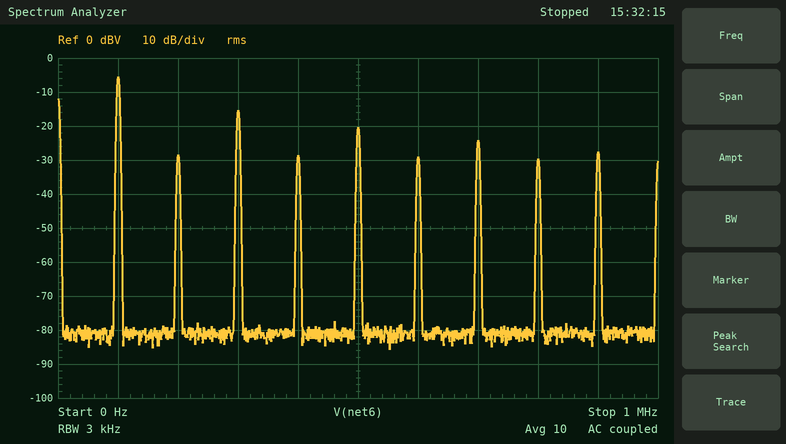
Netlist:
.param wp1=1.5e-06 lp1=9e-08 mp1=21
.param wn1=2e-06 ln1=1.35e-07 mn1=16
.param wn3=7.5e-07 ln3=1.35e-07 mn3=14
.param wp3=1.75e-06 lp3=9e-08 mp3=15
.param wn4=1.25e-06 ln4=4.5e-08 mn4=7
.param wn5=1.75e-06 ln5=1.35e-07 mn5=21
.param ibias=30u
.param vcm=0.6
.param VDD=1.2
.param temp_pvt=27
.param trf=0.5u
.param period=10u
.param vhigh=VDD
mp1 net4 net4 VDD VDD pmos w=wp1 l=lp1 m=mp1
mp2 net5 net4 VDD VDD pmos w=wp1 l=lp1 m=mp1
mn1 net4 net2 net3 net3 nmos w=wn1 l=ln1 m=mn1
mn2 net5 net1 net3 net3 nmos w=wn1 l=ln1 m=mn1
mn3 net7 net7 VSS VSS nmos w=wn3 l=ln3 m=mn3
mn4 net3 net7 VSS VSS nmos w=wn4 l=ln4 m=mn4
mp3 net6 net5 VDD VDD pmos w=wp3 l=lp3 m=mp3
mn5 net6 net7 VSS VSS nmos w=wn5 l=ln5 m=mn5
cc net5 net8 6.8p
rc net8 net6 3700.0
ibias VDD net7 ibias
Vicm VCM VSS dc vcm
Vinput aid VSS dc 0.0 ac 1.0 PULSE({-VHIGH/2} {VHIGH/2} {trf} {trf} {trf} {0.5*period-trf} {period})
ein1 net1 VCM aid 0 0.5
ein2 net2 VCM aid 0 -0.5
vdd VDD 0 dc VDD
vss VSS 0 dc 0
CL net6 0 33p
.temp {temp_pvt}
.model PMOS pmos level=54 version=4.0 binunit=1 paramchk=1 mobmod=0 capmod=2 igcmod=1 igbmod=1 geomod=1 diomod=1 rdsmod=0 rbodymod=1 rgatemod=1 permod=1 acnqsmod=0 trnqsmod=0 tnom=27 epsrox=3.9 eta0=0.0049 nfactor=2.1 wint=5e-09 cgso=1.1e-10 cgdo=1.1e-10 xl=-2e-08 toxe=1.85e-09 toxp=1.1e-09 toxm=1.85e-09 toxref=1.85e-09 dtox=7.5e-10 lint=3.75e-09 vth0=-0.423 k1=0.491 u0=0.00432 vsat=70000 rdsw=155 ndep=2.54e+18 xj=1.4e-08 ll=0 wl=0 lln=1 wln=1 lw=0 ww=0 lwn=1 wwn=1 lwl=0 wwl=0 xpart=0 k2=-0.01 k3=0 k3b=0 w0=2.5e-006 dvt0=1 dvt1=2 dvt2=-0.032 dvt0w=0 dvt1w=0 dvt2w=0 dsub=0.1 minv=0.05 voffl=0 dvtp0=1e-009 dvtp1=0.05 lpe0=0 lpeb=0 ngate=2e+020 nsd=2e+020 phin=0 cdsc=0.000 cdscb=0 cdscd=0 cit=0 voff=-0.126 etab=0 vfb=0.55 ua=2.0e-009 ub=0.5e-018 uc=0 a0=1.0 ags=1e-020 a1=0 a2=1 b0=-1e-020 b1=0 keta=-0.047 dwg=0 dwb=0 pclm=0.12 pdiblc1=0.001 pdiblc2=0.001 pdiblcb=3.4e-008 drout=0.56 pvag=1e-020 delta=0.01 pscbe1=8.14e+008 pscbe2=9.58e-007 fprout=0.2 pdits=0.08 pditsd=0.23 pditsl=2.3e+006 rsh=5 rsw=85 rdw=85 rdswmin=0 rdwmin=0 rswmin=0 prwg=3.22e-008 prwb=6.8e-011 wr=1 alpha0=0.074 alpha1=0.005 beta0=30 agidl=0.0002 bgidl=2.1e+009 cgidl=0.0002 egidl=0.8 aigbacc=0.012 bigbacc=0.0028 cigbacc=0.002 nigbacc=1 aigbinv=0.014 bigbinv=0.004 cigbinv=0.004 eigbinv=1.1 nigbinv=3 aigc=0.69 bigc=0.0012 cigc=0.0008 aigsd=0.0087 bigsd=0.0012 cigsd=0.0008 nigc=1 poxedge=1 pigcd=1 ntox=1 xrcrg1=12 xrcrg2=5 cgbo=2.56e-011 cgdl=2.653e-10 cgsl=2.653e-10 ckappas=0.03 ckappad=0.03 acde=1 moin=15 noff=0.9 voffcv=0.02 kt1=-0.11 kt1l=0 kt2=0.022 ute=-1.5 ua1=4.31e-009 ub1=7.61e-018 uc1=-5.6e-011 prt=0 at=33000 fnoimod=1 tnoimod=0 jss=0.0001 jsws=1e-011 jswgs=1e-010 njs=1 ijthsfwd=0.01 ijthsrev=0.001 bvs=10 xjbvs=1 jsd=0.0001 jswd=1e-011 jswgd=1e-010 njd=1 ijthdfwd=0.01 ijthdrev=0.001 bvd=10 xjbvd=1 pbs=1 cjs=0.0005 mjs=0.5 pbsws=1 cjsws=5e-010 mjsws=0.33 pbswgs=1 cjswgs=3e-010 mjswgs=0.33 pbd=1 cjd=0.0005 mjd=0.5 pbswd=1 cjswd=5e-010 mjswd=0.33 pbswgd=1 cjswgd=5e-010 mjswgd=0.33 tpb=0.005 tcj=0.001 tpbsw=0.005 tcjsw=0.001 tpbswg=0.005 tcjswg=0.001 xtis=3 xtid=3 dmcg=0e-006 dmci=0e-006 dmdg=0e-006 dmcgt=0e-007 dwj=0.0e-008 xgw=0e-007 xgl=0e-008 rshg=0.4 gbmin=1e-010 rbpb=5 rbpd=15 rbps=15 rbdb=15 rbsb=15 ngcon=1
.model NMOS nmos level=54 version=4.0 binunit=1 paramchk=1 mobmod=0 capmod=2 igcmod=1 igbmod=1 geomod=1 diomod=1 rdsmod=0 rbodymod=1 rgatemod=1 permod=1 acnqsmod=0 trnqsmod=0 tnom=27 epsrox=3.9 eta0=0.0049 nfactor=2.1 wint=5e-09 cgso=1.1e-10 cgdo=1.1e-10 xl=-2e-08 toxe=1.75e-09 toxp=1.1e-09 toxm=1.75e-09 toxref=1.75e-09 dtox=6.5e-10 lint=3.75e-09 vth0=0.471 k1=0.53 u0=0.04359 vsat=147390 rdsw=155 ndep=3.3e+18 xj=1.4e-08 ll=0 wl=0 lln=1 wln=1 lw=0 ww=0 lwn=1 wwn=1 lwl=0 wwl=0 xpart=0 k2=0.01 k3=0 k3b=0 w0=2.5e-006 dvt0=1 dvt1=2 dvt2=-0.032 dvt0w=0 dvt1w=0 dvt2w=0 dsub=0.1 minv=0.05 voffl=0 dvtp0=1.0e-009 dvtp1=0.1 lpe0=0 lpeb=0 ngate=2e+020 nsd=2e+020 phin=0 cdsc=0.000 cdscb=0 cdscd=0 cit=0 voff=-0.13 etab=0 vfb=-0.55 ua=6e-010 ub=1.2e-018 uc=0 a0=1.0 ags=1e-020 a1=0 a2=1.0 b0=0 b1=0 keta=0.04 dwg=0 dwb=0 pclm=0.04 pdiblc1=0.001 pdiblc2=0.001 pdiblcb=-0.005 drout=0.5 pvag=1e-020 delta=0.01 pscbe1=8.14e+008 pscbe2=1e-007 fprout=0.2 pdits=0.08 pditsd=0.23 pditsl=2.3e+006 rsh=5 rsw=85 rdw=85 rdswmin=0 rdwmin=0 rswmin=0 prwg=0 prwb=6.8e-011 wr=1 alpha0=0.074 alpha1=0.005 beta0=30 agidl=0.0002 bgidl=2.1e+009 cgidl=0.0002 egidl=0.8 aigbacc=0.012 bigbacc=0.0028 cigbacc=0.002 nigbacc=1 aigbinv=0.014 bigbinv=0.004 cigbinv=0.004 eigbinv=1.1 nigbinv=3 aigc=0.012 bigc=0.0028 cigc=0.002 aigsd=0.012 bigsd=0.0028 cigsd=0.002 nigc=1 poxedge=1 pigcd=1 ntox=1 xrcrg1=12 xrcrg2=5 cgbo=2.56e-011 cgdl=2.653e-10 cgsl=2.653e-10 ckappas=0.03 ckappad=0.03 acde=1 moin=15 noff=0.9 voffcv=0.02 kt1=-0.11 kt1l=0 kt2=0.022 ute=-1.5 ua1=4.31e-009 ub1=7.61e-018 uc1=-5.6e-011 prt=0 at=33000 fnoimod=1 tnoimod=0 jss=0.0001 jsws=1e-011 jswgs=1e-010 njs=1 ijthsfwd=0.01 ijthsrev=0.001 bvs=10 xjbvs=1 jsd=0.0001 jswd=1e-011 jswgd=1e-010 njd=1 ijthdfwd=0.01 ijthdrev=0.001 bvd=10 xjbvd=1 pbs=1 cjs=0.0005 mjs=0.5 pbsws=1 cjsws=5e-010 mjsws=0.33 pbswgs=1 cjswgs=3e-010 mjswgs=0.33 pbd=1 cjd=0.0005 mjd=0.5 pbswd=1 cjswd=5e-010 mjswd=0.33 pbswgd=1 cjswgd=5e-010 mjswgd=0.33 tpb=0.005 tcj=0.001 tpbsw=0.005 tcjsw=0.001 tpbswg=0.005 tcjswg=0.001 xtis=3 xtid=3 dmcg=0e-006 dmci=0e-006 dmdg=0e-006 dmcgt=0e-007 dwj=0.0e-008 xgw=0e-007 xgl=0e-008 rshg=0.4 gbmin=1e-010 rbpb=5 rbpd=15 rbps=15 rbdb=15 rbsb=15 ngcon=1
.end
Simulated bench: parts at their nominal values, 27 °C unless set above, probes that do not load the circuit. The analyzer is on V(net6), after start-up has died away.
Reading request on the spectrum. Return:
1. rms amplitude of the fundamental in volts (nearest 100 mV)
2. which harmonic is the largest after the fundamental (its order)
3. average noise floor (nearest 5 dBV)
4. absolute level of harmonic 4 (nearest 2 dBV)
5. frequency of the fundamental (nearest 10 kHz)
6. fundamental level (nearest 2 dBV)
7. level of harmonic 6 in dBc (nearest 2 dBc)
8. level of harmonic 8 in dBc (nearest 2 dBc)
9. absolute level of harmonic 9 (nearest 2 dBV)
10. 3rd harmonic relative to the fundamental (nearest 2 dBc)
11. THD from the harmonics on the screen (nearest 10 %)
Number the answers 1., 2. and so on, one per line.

1. 500 mV
2. 3
3. -80 dBV
4. -28 dBV
5. 100 kHz
6. -6 dBV
7. -24 dBc
8. -24 dBc
9. -28 dBV
10. -10 dBc
11. 40 %
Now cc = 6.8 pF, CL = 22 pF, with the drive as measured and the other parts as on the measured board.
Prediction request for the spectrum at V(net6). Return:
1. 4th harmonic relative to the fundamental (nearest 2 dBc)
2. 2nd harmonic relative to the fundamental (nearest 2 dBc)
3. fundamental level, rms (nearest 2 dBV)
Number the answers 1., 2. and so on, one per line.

1. -26 dBc
2. -26 dBc
3. -6 dBV
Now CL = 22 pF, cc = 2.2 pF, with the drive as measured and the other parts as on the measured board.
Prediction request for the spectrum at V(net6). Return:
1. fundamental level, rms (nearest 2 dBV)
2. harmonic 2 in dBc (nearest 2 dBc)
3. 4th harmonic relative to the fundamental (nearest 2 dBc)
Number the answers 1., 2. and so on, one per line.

1. -6 dBV
2. -28 dBc
3. -28 dBc
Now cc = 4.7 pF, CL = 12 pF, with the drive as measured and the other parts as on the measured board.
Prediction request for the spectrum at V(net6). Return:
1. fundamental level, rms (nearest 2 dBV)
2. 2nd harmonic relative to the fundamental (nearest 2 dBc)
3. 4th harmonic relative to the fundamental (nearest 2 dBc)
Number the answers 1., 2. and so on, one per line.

1. -6 dBV
2. -30 dBc
3. -30 dBc
